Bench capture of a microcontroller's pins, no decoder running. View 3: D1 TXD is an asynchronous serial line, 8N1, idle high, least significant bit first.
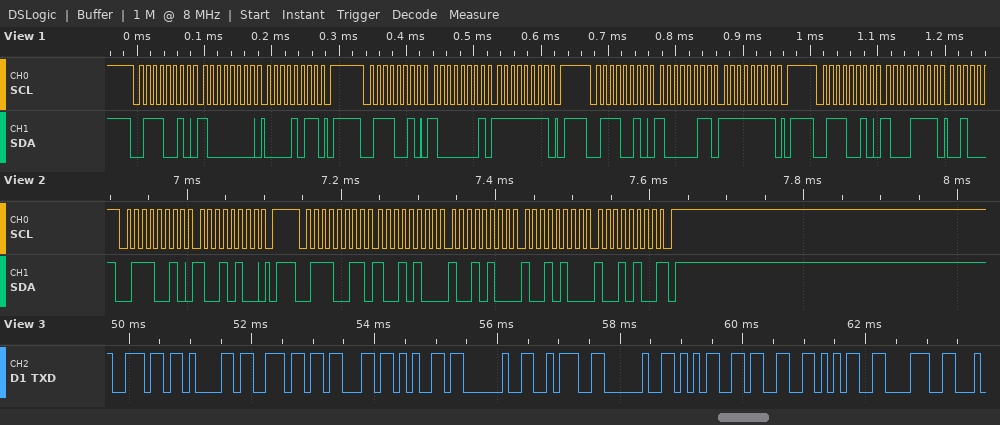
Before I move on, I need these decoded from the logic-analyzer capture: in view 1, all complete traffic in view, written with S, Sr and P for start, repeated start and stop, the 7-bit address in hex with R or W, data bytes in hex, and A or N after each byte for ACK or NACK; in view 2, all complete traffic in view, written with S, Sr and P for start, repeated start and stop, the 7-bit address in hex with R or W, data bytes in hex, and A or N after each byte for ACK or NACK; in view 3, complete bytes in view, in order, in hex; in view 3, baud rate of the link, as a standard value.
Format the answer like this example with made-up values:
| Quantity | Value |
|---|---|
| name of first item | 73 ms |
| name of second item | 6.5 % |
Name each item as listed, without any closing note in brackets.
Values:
| Quantity | Value |
|---|---|
| in view 1, all complete traffic in view, written with S, Sr and P for start, repeated start and stop, the 7-bit address in hex with R or W, data bytes in hex, and A or N after each byte for ACK or NACK | S 39W A 80 A 0B A P S 39W A 81 A FF A P S 39W A 83 A FF A P S 39W A 8F A |
| in view 2, all complete traffic in view, written with S, Sr and P for start, repeated start and stop, the 7-bit address in hex with R or W, data bytes in hex, and A or N after each byte for ACK or NACK | S 39W A 94 A P S 39R A 94 A 94 A 94 A 94 N P |
| in view 3, complete bytes in view, in order, in hex | 6E 61 6E 63 65 20 3A 20 35 33 35 38 |
| in view 3, baud rate of the link, as a standard value | 9600 baud |
